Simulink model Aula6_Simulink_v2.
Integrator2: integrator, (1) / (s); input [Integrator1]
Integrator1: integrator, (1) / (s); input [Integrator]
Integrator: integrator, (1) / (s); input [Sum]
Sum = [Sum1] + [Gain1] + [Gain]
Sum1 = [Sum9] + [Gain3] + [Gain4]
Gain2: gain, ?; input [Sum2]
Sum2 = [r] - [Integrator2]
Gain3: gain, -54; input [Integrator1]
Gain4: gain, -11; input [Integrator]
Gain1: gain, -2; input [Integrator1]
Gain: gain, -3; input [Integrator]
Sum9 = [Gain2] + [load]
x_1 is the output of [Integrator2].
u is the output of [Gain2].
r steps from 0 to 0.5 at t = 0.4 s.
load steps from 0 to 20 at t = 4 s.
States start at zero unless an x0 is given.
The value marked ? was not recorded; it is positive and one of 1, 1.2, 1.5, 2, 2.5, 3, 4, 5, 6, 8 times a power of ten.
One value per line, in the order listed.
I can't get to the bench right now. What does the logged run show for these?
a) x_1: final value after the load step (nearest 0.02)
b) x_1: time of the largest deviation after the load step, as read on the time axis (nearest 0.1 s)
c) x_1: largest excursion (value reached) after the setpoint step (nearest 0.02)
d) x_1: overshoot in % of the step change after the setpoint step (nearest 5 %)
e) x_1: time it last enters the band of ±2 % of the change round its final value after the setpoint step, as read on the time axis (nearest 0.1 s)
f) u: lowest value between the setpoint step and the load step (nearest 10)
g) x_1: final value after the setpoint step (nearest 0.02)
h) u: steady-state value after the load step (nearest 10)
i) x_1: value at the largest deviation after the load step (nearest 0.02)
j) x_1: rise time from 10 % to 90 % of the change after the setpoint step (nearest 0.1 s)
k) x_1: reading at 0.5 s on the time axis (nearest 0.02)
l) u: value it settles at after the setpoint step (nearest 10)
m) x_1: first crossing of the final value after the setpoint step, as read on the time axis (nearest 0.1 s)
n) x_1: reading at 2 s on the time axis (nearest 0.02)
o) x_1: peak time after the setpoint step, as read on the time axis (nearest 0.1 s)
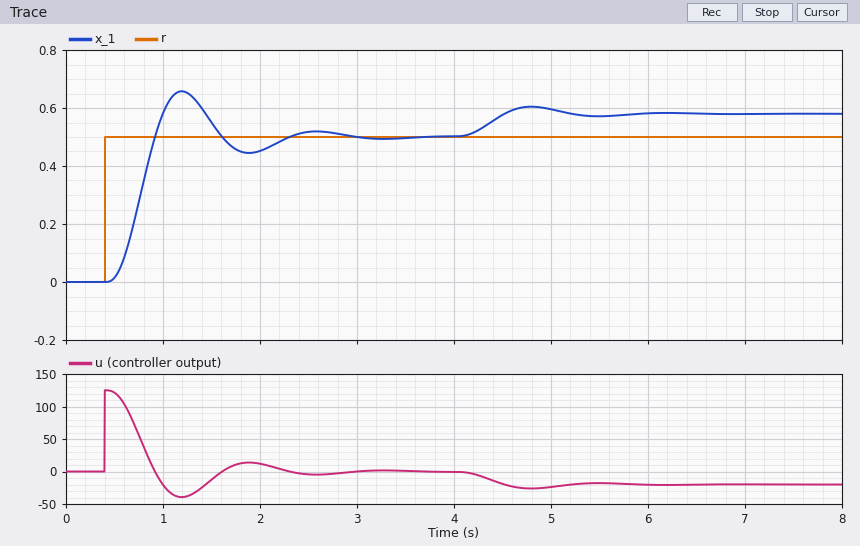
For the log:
0.58
4.8 s
0.66
30 %
2.8 s
-40
0.50
-20
0.60
0.3 s
0.02
0
0.9 s
0.46
1.2 s
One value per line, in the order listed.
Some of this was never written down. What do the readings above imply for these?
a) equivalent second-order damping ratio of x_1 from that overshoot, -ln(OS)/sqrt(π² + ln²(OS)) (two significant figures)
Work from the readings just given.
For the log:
0.36
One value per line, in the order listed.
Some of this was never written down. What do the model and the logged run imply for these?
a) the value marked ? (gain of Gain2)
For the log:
250
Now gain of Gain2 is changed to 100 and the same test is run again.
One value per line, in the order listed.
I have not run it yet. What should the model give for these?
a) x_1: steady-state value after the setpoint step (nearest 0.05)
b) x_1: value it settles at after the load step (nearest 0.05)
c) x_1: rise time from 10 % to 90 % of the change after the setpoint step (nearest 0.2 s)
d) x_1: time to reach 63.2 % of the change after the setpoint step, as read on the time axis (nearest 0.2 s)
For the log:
0.50
0.70
0.8 s
1.0 s
